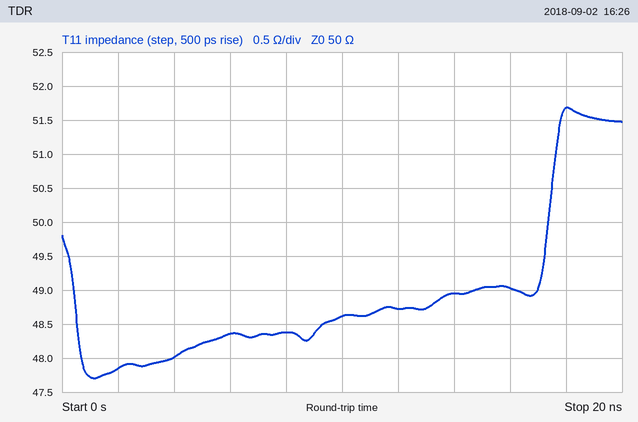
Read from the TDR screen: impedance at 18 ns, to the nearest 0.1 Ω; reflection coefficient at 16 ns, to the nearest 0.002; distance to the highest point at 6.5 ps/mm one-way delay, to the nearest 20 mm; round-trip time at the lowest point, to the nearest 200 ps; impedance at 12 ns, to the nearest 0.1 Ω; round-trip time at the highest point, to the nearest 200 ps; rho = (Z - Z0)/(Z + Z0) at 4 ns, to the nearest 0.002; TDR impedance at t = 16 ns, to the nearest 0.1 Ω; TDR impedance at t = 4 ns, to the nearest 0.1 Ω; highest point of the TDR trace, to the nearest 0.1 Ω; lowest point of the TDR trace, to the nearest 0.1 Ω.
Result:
51.7 Ω
-0.010
1.38 m
1.2 ns
48.7 Ω
18.0 ns
-0.020
49.0 Ω
48.0 Ω
51.7 Ω
47.7 Ω
